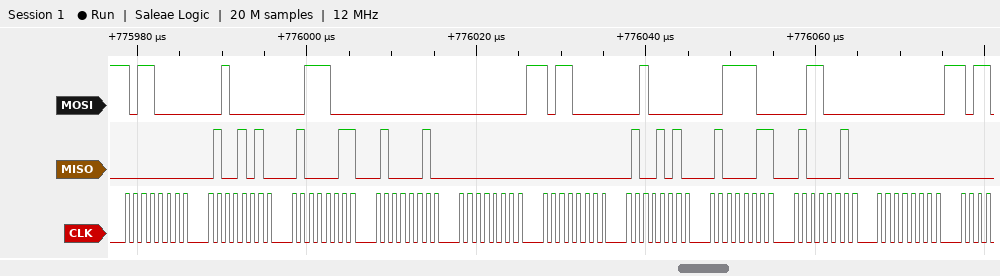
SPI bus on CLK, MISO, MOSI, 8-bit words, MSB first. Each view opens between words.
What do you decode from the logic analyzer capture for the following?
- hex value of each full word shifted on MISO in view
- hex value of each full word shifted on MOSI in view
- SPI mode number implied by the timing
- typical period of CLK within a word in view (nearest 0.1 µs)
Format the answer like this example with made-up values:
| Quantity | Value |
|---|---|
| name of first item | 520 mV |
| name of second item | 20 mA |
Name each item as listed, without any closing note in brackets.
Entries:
| Quantity | Value |
|---|---|
| hex value of each full word shifted on MISO in view | 00, 4A, 43, 42, 00, 00, 4A, 43, 42, 00 |
| hex value of each full word shifted on MOSI in view | B0, 20, 38, 00, 00, B0, 20, 3C, 30, 00 |
| SPI mode number implied by the timing | 0 |
| typical period of CLK within a word in view | 1 µs |
